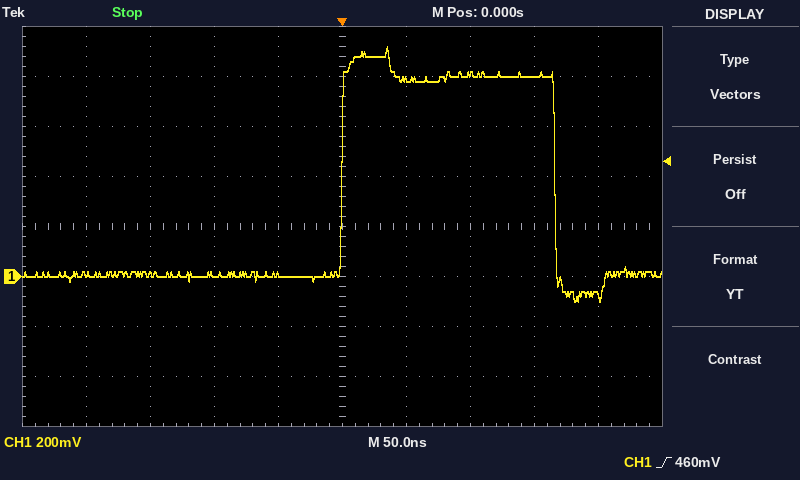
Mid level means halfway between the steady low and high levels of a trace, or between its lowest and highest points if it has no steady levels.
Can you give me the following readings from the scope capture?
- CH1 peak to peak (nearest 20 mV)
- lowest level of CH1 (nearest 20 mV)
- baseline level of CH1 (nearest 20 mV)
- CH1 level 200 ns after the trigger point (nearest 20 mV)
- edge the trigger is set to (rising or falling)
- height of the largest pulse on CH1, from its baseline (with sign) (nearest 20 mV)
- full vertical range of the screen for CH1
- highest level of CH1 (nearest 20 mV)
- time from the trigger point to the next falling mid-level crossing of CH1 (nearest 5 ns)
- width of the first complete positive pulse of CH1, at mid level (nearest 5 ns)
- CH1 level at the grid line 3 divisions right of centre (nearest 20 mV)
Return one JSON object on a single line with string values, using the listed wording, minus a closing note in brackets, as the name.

{"CH1 peak to peak": "1.02 V", "lowest level of CH1": "-100 mV", "baseline level of CH1": "0 mV", "CH1 level 200 ns after the trigger point": "-80 mV", "edge the trigger is set to": "rising", "height of the largest pulse on CH1, from its baseline (with sign)": "+920 mV", "full vertical range of the screen for CH1": "1.6 V", "highest level of CH1": "920 mV", "time from the trigger point to the next falling mid-level crossing of CH1": "165 ns", "width of the first complete positive pulse of CH1, at mid level": "165 ns", "CH1 level at the grid line 3 divisions right of centre": "800 mV"}
